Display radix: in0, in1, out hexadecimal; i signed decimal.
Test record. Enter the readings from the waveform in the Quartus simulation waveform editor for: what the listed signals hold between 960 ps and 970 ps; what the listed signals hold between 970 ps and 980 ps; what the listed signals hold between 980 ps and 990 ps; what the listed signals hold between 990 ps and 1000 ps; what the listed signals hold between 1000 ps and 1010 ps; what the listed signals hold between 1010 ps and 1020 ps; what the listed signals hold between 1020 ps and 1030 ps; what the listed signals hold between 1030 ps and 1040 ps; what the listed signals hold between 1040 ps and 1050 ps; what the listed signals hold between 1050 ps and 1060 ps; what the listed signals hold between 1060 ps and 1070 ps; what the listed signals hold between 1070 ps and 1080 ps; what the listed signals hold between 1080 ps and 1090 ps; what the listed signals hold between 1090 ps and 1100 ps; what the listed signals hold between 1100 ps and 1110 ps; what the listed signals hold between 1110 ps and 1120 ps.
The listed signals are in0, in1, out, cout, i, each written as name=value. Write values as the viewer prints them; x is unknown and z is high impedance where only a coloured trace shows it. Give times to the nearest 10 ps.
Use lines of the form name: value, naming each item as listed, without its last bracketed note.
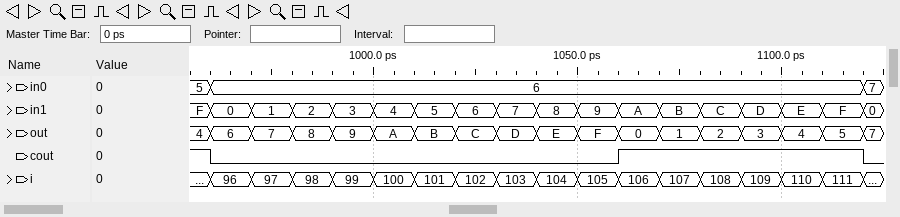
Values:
what the listed signals hold between 960 ps and 970 ps: in0=6, in1=0, out=6, cout=0, i=96
what the listed signals hold between 970 ps and 980 ps: in0=6, in1=1, out=7, cout=0, i=97
what the listed signals hold between 980 ps and 990 ps: in0=6, in1=2, out=8, cout=0, i=98
what the listed signals hold between 990 ps and 1000 ps: in0=6, in1=3, out=9, cout=0, i=99
what the listed signals hold between 1000 ps and 1010 ps: in0=6, in1=4, out=A, cout=0, i=100
what the listed signals hold between 1010 ps and 1020 ps: in0=6, in1=5, out=B, cout=0, i=101
what the listed signals hold between 1020 ps and 1030 ps: in0=6, in1=6, out=C, cout=0, i=102
what the listed signals hold between 1030 ps and 1040 ps: in0=6, in1=7, out=D, cout=0, i=103
what the listed signals hold between 1040 ps and 1050 ps: in0=6, in1=8, out=E, cout=0, i=104
what the listed signals hold between 1050 ps and 1060 ps: in0=6, in1=9, out=F, cout=0, i=105
what the listed signals hold between 1060 ps and 1070 ps: in0=6, in1=A, out=0, cout=1, i=106
what the listed signals hold between 1070 ps and 1080 ps: in0=6, in1=B, out=1, cout=1, i=107
what the listed signals hold between 1080 ps and 1090 ps: in0=6, in1=C, out=2, cout=1, i=108
what the listed signals hold between 1090 ps and 1100 ps: in0=6, in1=D, out=3, cout=1, i=109
what the listed signals hold between 1100 ps and 1110 ps: in0=6, in1=E, out=4, cout=1, i=110
what the listed signals hold between 1110 ps and 1120 ps: in0=6, in1=F, out=5, cout=1, i=111
